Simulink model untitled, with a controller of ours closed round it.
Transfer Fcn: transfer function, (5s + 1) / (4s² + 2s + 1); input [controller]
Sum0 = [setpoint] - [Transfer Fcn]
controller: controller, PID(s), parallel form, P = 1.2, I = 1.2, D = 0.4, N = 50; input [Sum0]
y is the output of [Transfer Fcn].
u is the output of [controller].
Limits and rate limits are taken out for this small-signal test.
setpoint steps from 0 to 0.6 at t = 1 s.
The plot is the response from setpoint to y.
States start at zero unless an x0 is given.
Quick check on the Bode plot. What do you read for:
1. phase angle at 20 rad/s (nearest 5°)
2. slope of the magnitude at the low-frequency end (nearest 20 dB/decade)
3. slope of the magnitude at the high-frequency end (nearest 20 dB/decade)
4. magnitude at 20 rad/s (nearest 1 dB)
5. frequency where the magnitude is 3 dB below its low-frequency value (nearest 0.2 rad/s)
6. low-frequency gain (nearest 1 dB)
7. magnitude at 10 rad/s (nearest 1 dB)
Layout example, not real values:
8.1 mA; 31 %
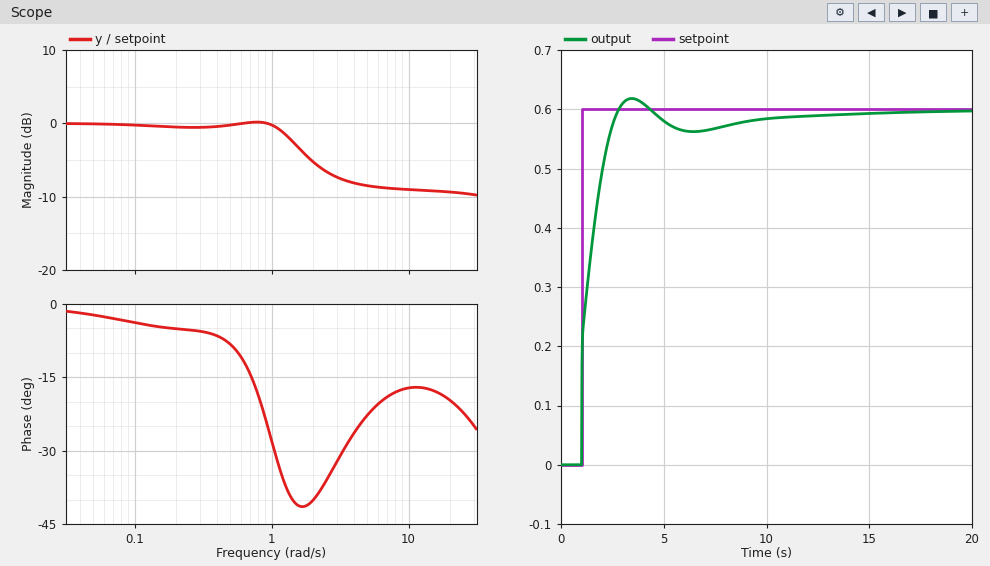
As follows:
-20°; 0 dB/decade; 0 dB/decade; -9 dB; 1.6 rad/s; 0 dB; -9 dB
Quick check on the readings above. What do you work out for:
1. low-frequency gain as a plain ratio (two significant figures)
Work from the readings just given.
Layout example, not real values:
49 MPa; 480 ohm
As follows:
1.0
